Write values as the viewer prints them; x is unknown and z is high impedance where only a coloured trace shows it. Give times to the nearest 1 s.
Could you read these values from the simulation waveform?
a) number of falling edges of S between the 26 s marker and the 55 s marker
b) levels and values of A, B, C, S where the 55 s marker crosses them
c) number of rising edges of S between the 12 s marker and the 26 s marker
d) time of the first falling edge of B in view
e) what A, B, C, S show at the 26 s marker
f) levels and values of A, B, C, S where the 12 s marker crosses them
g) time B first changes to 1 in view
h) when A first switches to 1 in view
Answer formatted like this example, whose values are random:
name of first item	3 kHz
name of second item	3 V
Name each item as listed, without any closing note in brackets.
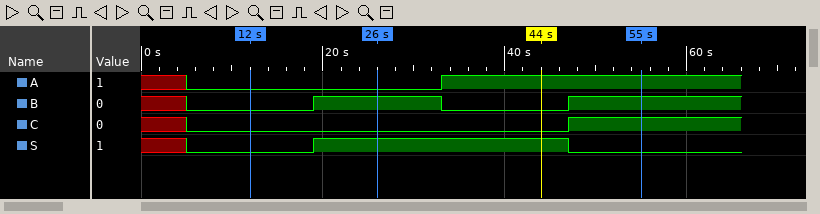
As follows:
number of falling edges of S between the 26 s marker and the 55 s marker	1
levels and values of A, B, C, S where the 55 s marker crosses them	A=1, B=1, C=1, S=0
number of rising edges of S between the 12 s marker and the 26 s marker	1
time of the first falling edge of B in view	33 s
what A, B, C, S show at the 26 s marker	A=0, B=1, C=0, S=1
levels and values of A, B, C, S where the 12 s marker crosses them	A=0, B=0, C=0, S=0
time B first changes to 1 in view	19 s
when A first switches to 1 in view	33 s
